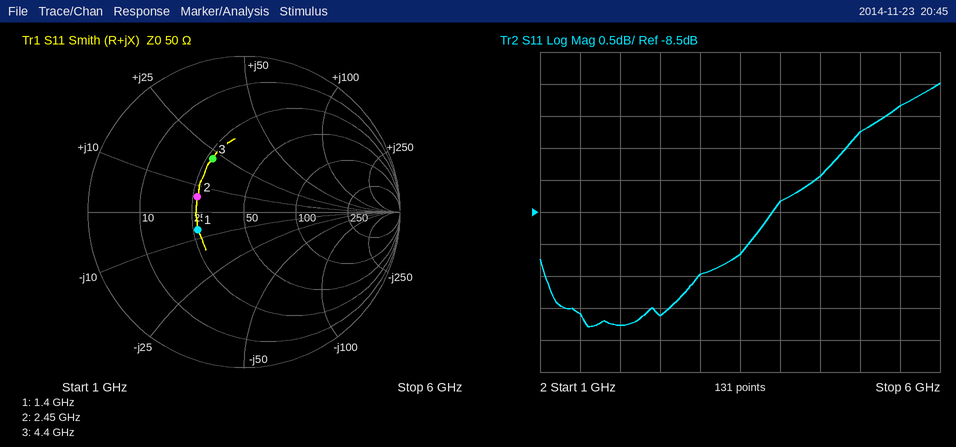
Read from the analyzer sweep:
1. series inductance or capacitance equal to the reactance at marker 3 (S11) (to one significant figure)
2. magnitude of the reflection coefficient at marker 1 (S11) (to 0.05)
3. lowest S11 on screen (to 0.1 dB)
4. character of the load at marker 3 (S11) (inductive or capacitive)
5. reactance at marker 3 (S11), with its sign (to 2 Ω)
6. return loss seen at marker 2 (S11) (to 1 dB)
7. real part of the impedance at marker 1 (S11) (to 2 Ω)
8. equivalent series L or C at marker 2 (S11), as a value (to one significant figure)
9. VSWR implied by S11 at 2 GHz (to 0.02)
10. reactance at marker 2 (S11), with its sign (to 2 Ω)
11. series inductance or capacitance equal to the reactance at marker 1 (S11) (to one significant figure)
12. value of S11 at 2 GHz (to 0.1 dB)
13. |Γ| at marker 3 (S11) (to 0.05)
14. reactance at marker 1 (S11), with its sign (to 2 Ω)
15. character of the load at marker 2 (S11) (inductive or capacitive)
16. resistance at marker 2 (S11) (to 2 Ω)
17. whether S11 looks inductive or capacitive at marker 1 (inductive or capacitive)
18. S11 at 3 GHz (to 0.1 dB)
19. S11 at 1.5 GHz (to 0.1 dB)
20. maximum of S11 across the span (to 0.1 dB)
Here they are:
800 pH
0.30
-10.3 dB
inductive
+22 Ω
10 dB
26 Ω
400 pH
1.88
+6 Ω
20 pF
-10.3 dB
0.40
-6 Ω
inductive
26 Ω
capacitive
-9.5 dB
-10.1 dB
-6.5 dB
